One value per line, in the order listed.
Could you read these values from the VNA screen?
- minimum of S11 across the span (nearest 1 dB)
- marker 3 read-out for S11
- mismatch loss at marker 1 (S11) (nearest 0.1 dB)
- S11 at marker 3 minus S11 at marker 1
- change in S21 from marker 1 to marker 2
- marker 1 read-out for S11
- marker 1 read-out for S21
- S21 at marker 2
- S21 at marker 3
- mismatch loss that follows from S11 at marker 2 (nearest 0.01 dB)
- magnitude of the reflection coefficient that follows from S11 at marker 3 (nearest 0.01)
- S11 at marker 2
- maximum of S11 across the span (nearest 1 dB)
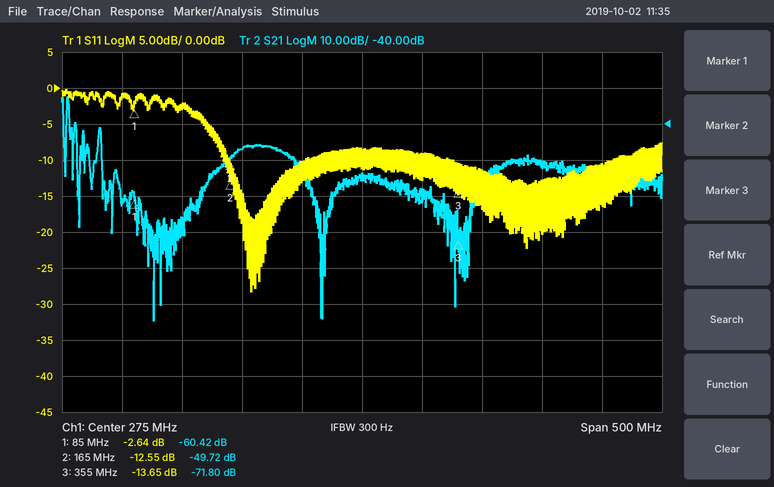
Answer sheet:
-28 dB
-13.65 dB
3.4 dB
-11.01 dB
10.70 dB
-2.64 dB
-60.42 dB
-49.72 dB
-71.80 dB
0.25 dB
0.21
-12.55 dB
0 dB
